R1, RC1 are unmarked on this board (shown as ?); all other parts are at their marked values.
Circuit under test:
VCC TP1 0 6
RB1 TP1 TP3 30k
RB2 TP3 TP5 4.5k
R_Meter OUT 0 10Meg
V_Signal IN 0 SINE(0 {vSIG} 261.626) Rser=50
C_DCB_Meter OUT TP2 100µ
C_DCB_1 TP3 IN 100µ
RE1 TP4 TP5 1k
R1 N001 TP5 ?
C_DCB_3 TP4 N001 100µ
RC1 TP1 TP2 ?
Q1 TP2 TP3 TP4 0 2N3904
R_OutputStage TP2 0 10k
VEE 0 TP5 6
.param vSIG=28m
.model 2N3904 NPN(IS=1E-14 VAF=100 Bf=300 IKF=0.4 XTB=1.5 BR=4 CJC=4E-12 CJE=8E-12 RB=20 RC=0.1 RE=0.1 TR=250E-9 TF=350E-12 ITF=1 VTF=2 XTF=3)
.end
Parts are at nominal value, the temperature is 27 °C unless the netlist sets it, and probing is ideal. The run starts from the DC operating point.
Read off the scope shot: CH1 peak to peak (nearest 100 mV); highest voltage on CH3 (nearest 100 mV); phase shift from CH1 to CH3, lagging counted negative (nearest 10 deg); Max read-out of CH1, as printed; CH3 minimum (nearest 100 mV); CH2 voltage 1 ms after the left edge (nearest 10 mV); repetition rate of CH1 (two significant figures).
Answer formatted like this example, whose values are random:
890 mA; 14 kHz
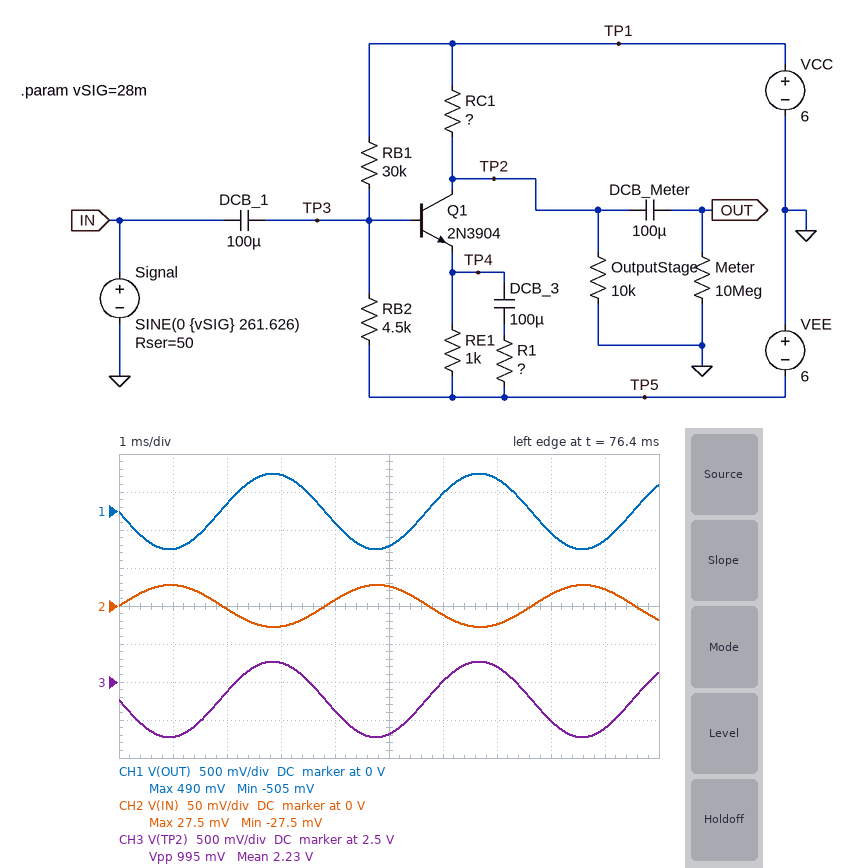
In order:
1.0 V; 2.8 V; 0 deg; 490 mV; 1.8 V; 30 mV; 260 Hz
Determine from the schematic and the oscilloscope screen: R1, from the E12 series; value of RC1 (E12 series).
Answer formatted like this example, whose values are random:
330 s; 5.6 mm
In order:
120 Ω; 3.3 kΩ
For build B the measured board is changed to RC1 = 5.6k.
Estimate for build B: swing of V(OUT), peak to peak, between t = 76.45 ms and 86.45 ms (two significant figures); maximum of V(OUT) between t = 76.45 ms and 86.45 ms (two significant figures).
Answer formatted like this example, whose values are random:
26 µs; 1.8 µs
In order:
1.4 V; 710 mV
